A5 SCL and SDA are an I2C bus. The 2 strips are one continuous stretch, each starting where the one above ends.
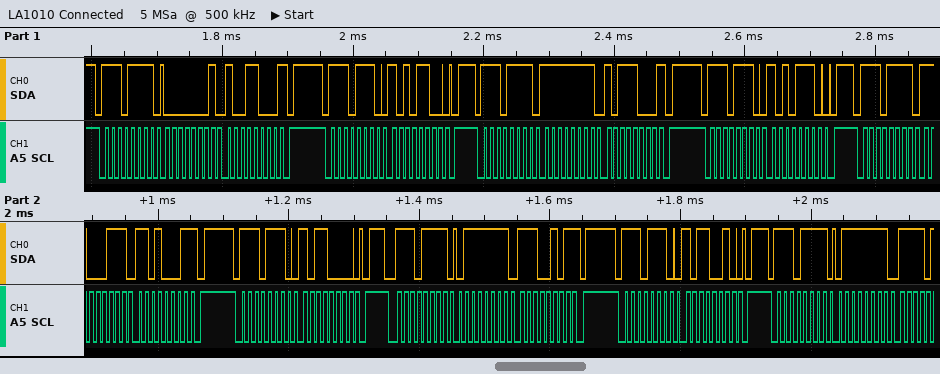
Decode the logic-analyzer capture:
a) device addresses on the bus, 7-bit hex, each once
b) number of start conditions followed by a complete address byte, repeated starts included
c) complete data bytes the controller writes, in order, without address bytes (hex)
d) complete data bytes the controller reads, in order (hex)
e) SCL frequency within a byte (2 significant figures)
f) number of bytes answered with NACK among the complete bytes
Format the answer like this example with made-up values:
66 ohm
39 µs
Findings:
0x77
9
AC AE B0 B2
01 98 FF B8 C7 D1 7F E5 7F
100 kHz
4
